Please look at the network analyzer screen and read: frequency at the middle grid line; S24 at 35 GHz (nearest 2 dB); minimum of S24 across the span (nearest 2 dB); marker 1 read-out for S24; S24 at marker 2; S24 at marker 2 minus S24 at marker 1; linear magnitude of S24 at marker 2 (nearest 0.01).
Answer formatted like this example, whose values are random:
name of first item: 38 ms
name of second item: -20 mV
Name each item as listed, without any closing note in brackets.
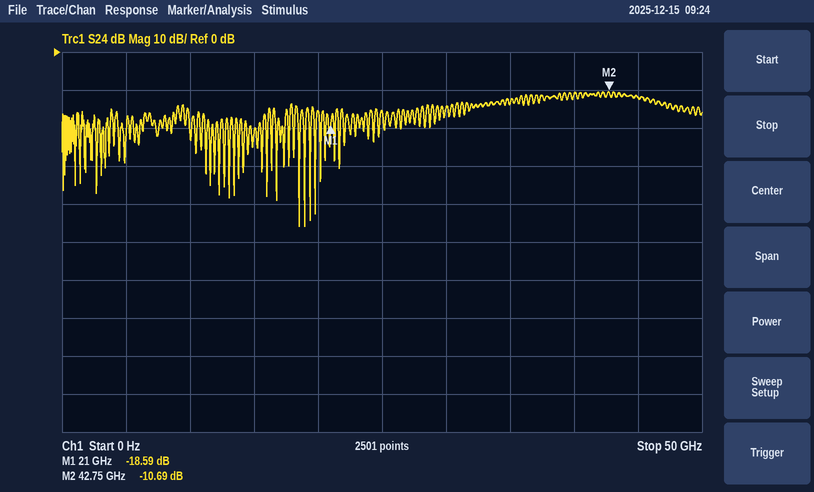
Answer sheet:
frequency at the middle grid line: 25 GHz
S24 at 35 GHz: -14 dB
minimum of S24 across the span: -46 dB
marker 1 read-out for S24: -18.59 dB
S24 at marker 2: -10.69 dB
S24 at marker 2 minus S24 at marker 1: 7.90 dB
linear magnitude of S24 at marker 2: 0.29
